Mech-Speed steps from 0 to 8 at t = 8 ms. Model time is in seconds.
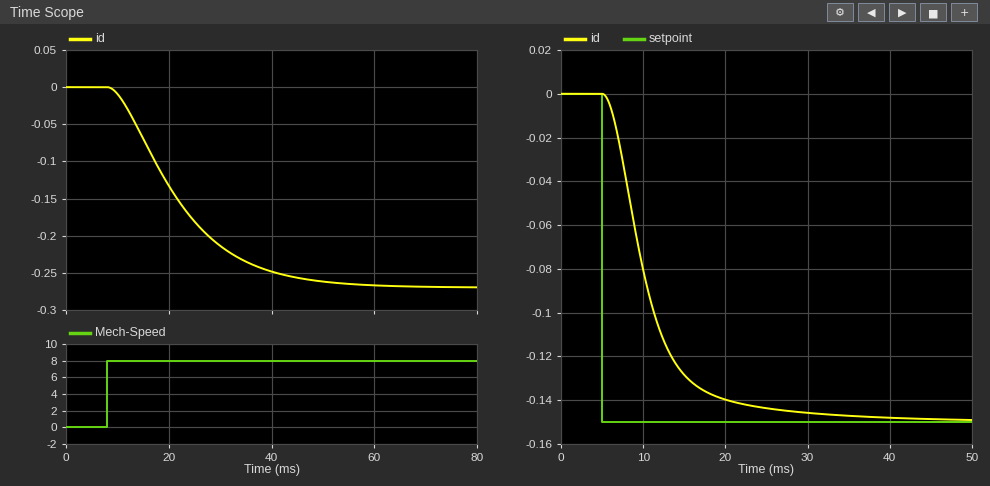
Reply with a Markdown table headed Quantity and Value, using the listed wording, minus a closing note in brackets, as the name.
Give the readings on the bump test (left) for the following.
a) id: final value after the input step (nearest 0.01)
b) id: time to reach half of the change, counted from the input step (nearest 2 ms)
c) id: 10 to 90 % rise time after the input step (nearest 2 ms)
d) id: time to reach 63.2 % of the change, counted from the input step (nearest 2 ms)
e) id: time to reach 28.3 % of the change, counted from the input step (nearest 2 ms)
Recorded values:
| Quantity | Value |
|---|---|
| id: final value after the input step | -0.27 |
| id: time to reach half of the change, counted from the input step | 12 ms |
| id: 10 to 90 % rise time after the input step | 26 ms |
| id: time to reach 63.2 % of the change, counted from the input step | 16 ms |
| id: time to reach 28.3 % of the change, counted from the input step | 8 ms |
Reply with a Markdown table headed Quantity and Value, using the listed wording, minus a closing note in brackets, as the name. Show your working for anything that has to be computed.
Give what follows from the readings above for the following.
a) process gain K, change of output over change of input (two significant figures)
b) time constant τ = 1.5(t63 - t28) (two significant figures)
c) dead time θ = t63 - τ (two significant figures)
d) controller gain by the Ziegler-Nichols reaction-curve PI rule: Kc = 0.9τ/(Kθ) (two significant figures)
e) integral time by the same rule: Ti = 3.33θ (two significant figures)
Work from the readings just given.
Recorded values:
| Quantity | Value |
|---|---|
| process gain K, change of output over change of input | (-0.27 - 0) / 8 = -0.034 |
| time constant τ = 1.5(t63 - t28) | 1.5 × (16 - 8) = 12 ms |
| dead time θ = t63 - τ | 16 - 12 = 4.0 ms |
| controller gain by the Ziegler-Nichols reaction-curve PI rule: Kc = 0.9τ/(Kθ) | 0.9 × 12 / (-0.034 × 4) = -79 |
| integral time by the same rule: Ti = 3.33θ | 3.33 × 4 = 13 ms |
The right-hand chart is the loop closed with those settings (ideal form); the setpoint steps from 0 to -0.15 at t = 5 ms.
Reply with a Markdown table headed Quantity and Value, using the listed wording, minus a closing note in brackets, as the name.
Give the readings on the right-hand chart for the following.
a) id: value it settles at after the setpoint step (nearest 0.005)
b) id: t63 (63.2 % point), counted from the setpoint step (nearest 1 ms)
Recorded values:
| Quantity | Value |
|---|---|
| id: value it settles at after the setpoint step | -0.150 |
| id: t63 (63.2 % point), counted from the setpoint step | 6 ms |
